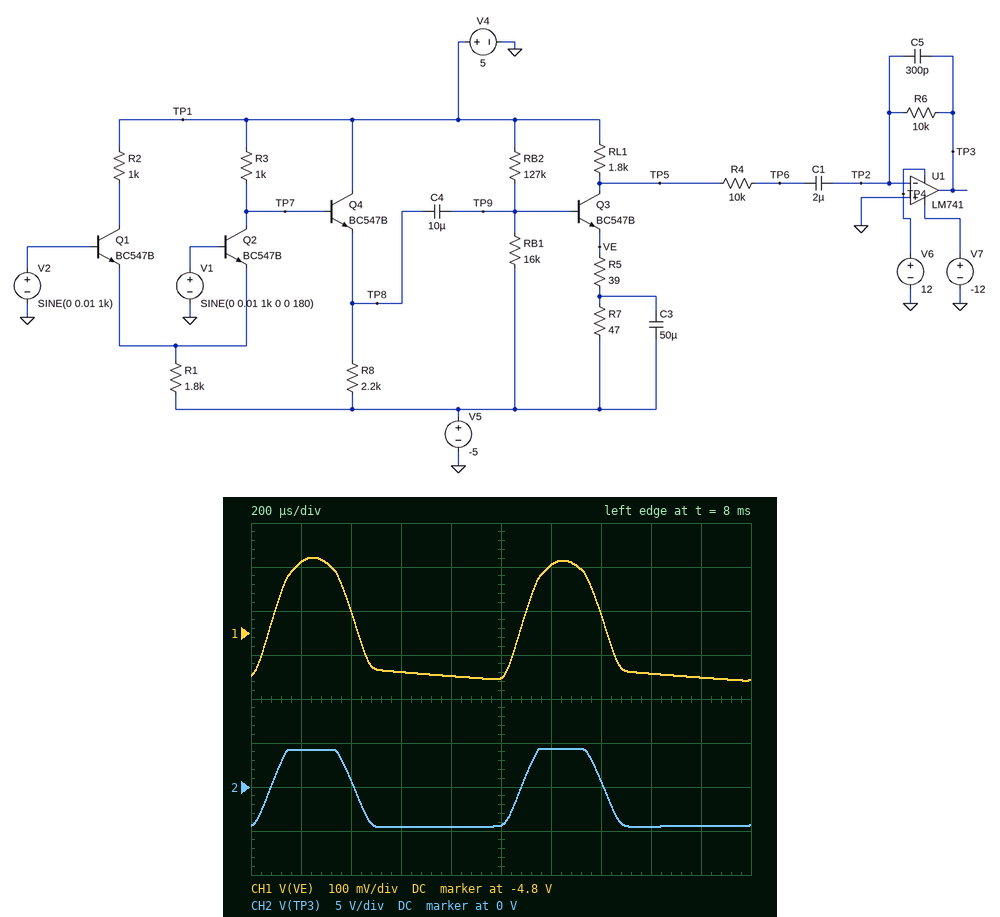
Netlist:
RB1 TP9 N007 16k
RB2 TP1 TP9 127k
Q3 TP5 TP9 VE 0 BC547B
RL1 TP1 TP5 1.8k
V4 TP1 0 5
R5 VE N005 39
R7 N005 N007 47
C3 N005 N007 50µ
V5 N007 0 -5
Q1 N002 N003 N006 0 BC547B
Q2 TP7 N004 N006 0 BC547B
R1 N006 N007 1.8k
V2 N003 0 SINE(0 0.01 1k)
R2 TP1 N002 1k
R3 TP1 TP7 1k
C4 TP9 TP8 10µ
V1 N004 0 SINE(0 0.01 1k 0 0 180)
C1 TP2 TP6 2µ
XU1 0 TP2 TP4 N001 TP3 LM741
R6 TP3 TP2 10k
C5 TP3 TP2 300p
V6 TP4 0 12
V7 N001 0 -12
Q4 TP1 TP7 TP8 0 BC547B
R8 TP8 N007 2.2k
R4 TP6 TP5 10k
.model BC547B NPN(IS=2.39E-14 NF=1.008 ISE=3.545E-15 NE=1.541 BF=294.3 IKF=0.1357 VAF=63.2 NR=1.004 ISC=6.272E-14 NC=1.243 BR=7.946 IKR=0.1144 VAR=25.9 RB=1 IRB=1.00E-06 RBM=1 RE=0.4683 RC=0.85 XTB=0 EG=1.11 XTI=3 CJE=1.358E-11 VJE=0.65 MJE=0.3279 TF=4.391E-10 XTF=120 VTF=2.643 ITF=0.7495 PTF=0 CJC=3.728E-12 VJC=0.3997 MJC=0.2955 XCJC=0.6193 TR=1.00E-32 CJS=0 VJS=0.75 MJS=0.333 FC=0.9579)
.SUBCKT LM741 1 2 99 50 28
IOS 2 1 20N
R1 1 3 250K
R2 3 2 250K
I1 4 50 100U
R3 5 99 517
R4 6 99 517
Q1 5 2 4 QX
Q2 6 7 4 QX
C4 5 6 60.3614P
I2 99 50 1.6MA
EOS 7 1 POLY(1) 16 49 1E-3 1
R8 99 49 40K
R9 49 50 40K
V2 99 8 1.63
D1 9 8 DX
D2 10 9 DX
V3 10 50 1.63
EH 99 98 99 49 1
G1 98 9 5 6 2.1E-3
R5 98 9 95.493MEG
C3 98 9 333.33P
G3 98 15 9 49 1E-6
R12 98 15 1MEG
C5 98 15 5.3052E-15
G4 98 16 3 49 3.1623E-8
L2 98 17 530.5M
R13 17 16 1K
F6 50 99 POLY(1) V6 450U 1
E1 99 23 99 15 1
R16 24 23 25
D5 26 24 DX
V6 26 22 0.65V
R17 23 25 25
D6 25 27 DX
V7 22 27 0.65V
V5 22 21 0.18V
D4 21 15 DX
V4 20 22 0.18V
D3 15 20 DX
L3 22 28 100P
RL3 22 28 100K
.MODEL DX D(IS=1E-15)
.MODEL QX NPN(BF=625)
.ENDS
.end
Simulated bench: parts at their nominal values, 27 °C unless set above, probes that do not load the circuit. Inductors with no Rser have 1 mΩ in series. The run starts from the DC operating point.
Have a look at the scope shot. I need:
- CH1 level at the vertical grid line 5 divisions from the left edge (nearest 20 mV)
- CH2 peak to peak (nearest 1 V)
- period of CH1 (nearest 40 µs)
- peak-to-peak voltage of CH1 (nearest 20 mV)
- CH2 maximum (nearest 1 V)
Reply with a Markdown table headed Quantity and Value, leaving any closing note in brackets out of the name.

| Quantity | Value |
|---|---|
| CH1 level at the vertical grid line 5 divisions from the left edge | -4.90 V |
| CH2 peak to peak | 9 V |
| period of CH1 | 1.00 ms |
| peak-to-peak voltage of CH1 | 280 mV |
| CH2 maximum | 4 V |
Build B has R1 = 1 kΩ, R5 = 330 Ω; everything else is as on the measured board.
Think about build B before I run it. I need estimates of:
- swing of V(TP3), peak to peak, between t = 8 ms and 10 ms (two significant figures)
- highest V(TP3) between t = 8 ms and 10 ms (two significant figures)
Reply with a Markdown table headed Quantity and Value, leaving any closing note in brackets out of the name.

| Quantity | Value |
|---|---|
| swing of V(TP3), peak to peak, between t = 8 ms and 10 ms | 4.9 V |
| highest V(TP3) between t = 8 ms and 10 ms | 3.1 V |
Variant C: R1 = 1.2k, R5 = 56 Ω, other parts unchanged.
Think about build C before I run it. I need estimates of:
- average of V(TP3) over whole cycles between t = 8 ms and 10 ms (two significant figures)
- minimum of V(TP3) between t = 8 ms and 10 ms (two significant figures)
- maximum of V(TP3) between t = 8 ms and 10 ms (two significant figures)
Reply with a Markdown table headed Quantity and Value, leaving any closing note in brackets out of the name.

| Quantity | Value |
|---|---|
| average of V(TP3) over whole cycles between t = 8 ms and 10 ms | -1.3 V |
| minimum of V(TP3) between t = 8 ms and 10 ms | -4.2 V |
| maximum of V(TP3) between t = 8 ms and 10 ms | 4.7 V |
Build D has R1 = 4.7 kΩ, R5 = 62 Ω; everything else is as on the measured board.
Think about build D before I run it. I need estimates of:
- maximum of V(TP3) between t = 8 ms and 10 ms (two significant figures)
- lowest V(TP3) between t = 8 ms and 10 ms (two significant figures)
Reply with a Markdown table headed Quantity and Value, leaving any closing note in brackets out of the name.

| Quantity | Value |
|---|---|
| maximum of V(TP3) between t = 8 ms and 10 ms | 3.5 V |
| lowest V(TP3) between t = 8 ms and 10 ms | -3.2 V |
